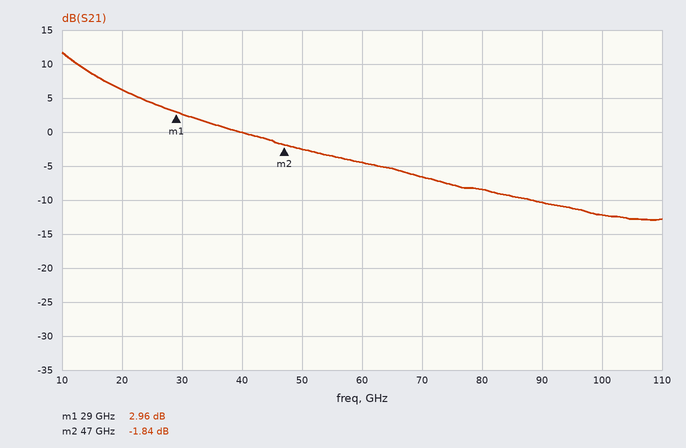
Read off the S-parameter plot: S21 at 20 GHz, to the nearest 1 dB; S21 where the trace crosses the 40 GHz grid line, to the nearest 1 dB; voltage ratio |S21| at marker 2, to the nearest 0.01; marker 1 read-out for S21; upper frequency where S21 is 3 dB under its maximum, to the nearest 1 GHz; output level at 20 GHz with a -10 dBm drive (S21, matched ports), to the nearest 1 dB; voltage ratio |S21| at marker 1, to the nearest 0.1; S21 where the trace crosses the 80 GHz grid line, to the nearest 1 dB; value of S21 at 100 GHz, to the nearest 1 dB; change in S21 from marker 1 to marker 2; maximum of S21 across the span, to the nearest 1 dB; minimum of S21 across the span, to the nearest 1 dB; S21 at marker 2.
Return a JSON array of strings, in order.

["6 dB", "0 dB", "0.81", "2.96 dB", "15 GHz", "-4 dBm", "1.4", "-8 dB", "-12 dB", "-4.80 dB", "12 dB", "-13 dB", "-1.84 dB"]
